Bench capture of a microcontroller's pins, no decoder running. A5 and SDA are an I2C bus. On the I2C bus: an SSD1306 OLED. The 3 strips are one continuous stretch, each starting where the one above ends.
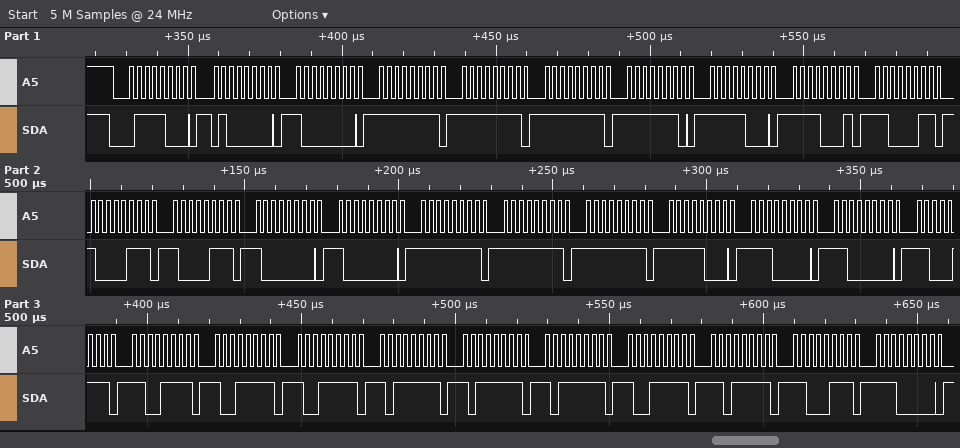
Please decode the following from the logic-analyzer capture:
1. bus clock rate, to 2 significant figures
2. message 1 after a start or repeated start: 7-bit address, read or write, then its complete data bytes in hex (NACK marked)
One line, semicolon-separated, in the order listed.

400 kHz; 0x3C write: 40 80 FF FF FF FE F8 F1 C3 87 87 80 80 FF FF FF F8 E0 C0 C7 CF 9F 9F BF BF BF 9F DF C7 E0
